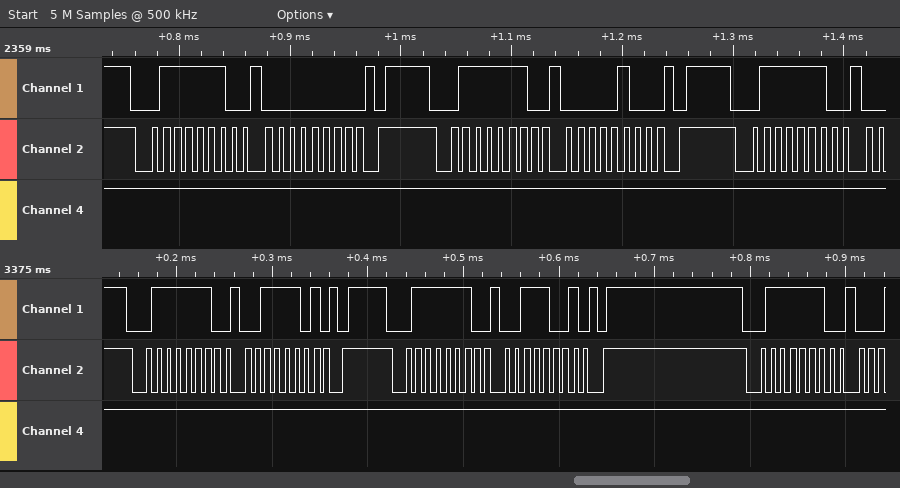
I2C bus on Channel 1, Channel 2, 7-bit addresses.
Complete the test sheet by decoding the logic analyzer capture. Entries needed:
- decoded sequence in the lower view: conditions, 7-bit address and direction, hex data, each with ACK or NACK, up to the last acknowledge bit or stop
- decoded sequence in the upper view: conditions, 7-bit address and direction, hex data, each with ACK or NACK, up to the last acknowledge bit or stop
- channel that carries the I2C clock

start, address 3F write ACK, 3D ACK, stop, start, address 3F write ACK, 39 ACK, stop, start, address 3F write ACK
start, address 3F write ACK, 00 ACK, stop, start, address 3F write ACK, 04 ACK, stop, start, address 3F write ACK
Channel 2
